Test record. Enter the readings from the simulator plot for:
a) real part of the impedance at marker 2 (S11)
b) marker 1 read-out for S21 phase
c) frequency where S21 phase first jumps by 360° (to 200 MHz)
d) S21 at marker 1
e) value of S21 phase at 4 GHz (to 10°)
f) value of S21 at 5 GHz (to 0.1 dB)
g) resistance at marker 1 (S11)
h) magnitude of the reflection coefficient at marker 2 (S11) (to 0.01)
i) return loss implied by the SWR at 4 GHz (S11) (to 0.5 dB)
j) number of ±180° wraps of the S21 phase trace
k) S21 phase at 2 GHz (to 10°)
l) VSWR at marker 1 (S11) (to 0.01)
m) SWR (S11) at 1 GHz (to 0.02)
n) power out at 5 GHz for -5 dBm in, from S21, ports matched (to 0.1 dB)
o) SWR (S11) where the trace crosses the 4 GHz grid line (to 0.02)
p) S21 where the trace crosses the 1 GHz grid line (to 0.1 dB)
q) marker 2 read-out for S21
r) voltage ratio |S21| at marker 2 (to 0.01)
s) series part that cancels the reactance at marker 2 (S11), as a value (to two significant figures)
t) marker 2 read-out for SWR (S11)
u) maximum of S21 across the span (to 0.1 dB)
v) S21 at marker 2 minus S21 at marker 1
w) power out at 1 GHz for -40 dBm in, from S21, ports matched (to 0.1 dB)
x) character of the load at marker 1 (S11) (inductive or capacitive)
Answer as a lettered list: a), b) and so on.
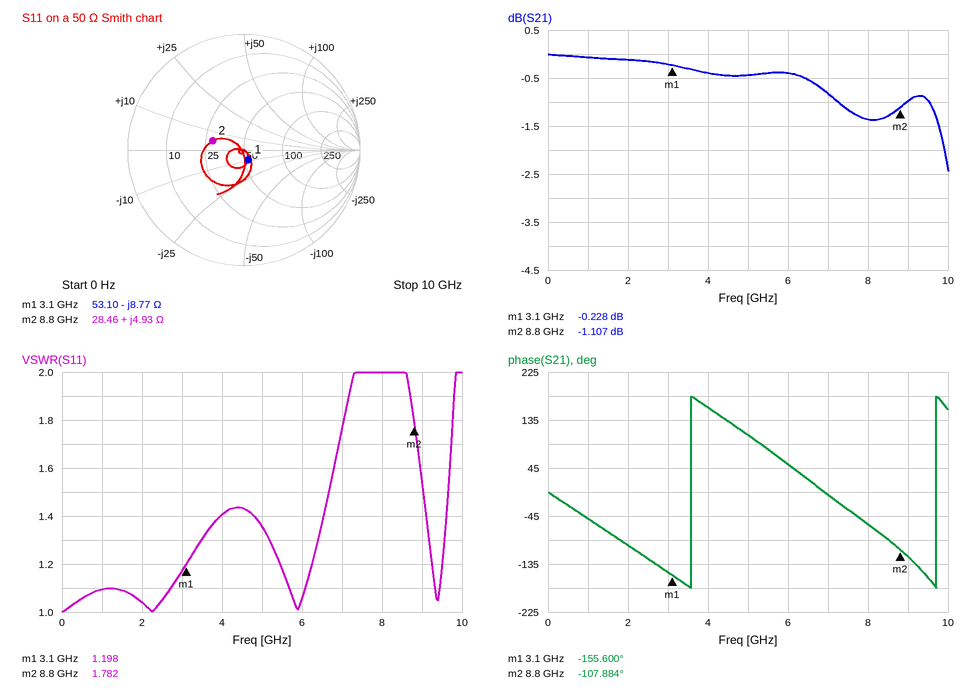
a) 28.46 Ω
b) -155.600°
c) 3.6 GHz
d) -0.228 dB
e) 160°
f) -0.4 dB
g) 53.10 Ω
h) 0.28
i) 15.5 dB
j) 2
k) -100°
l) 1.20
m) 1.10
n) -5.4 dBm
o) 1.40
p) -0.1 dB
q) -1.107 dB
r) 0.88
s) 3.7 pF
t) 1.782
u) 0.0 dB
v) -0.879 dB
w) -40.1 dBm
x) capacitive
